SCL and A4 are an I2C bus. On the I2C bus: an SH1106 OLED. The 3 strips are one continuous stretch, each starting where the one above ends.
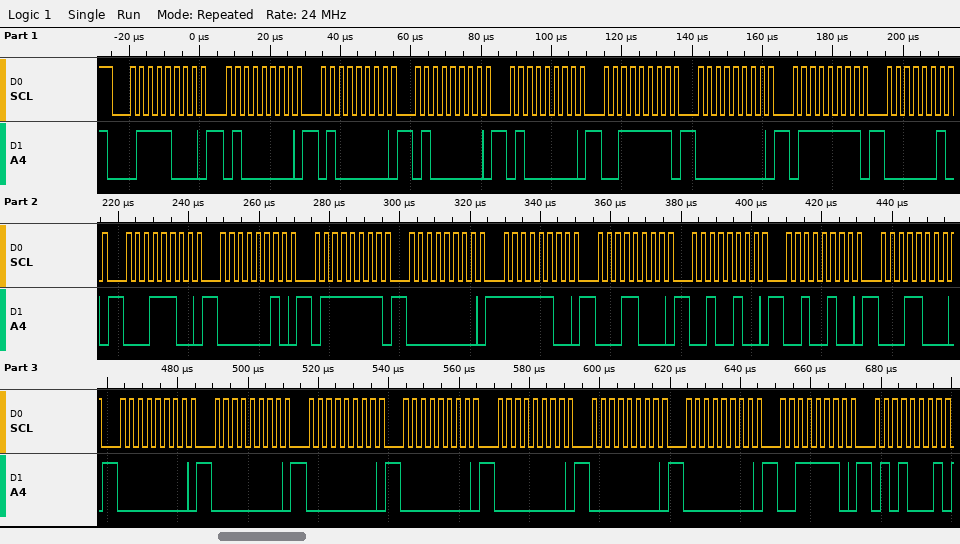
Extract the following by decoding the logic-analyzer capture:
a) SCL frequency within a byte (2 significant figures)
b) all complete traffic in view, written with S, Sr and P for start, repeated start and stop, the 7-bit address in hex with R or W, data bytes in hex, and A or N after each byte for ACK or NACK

400 kHz
S 3CW A 40 A 40 A 40 A 40 A 3F A 00 A 7F A 02 A 1C A 02 A 7F A 00 A FC A 18 A 24 A 24 A 18 A 00 A 00 A 00 A 00 A 00 A 00 A 00 A 3E A 51 A
